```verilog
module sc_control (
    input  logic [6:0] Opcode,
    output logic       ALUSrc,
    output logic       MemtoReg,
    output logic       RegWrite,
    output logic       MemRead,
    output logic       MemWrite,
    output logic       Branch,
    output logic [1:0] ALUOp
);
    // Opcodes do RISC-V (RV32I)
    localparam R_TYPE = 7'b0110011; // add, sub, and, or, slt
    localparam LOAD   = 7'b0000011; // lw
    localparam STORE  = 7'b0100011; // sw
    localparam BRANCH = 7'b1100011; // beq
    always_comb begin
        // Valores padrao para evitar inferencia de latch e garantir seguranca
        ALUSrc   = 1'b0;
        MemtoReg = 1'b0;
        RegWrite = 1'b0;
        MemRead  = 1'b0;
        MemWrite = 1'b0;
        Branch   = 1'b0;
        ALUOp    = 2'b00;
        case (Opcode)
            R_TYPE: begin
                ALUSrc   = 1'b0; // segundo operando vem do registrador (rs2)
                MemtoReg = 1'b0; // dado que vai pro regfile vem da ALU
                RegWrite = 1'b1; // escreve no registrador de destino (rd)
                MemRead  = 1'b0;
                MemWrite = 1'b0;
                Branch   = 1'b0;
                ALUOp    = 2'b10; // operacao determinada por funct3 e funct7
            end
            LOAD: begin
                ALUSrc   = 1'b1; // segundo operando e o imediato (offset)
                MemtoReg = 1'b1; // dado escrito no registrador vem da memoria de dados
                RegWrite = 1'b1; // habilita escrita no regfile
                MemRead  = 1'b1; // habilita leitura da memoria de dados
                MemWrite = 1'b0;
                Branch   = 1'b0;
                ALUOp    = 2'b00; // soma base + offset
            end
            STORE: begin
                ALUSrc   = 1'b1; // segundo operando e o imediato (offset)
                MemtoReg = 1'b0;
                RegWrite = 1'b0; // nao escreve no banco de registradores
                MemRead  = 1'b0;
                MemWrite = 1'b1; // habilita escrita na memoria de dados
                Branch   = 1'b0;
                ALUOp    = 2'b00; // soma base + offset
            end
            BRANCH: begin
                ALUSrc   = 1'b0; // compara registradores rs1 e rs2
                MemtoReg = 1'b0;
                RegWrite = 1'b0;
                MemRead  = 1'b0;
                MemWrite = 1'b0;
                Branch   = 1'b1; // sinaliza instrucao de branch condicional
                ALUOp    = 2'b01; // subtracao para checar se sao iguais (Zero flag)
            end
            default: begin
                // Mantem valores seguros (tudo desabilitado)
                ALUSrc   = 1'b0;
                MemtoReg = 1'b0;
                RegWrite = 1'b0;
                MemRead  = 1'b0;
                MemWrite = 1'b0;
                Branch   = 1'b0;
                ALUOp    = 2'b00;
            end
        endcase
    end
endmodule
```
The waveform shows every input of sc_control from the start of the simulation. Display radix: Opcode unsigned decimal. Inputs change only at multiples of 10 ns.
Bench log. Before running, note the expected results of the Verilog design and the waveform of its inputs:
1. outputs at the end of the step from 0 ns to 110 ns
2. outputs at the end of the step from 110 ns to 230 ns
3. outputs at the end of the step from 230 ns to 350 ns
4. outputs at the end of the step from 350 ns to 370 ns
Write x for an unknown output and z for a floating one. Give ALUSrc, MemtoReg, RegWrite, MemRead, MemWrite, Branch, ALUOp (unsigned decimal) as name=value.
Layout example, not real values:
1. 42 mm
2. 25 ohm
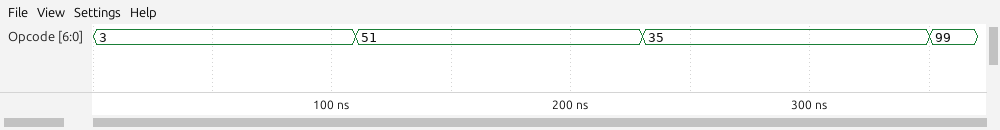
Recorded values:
1. ALUSrc=1, MemtoReg=1, RegWrite=1, MemRead=1, MemWrite=0, Branch=0, ALUOp=0
2. ALUSrc=0, MemtoReg=0, RegWrite=1, MemRead=0, MemWrite=0, Branch=0, ALUOp=2
3. ALUSrc=1, MemtoReg=0, RegWrite=0, MemRead=0, MemWrite=1, Branch=0, ALUOp=0
4. ALUSrc=0, MemtoReg=0, RegWrite=0, MemRead=0, MemWrite=0, Branch=1, ALUOp=1
